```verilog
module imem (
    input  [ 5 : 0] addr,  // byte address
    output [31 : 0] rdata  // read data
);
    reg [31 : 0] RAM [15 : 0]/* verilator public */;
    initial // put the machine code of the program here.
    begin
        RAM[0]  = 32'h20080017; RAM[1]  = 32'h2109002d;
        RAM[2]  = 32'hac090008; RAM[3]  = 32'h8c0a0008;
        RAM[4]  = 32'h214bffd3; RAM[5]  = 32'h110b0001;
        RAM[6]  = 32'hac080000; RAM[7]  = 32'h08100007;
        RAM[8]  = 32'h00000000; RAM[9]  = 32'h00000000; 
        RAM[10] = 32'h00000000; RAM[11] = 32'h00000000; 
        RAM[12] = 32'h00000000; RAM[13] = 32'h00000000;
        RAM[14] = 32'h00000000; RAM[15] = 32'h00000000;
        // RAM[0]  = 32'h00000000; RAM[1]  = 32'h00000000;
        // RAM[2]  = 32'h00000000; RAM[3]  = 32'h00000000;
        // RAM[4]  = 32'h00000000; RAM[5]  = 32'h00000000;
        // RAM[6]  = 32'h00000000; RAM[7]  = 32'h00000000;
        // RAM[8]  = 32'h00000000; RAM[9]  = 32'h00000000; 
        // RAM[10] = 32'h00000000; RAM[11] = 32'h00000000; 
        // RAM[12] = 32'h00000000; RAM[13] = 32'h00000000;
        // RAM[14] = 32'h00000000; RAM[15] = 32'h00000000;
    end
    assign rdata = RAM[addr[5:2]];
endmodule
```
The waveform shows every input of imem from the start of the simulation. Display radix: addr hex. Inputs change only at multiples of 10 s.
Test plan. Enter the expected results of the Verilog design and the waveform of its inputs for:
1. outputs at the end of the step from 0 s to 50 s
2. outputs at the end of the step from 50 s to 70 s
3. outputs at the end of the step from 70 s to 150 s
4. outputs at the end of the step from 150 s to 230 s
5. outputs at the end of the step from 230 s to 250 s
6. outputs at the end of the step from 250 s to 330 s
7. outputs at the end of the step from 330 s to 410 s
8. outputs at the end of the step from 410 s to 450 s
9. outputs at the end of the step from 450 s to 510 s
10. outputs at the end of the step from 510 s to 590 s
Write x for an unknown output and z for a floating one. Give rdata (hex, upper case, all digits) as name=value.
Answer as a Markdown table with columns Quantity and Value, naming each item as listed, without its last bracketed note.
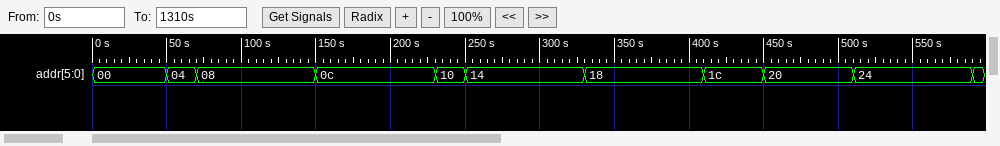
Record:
| Quantity | Value |
|---|---|
| outputs at the end of the step from 0 s to 50 s | rdata=20080017 |
| outputs at the end of the step from 50 s to 70 s | rdata=2109002D |
| outputs at the end of the step from 70 s to 150 s | rdata=AC090008 |
| outputs at the end of the step from 150 s to 230 s | rdata=8C0A0008 |
| outputs at the end of the step from 230 s to 250 s | rdata=214BFFD3 |
| outputs at the end of the step from 250 s to 330 s | rdata=110B0001 |
| outputs at the end of the step from 330 s to 410 s | rdata=AC080000 |
| outputs at the end of the step from 410 s to 450 s | rdata=08100007 |
| outputs at the end of the step from 450 s to 510 s | rdata=00000000 |
| outputs at the end of the step from 510 s to 590 s | rdata=00000000 |
